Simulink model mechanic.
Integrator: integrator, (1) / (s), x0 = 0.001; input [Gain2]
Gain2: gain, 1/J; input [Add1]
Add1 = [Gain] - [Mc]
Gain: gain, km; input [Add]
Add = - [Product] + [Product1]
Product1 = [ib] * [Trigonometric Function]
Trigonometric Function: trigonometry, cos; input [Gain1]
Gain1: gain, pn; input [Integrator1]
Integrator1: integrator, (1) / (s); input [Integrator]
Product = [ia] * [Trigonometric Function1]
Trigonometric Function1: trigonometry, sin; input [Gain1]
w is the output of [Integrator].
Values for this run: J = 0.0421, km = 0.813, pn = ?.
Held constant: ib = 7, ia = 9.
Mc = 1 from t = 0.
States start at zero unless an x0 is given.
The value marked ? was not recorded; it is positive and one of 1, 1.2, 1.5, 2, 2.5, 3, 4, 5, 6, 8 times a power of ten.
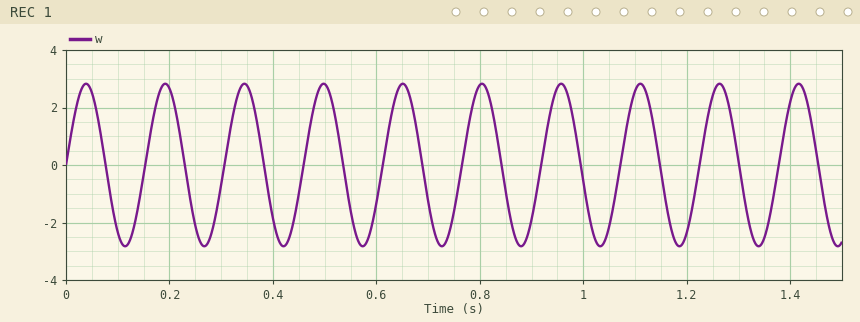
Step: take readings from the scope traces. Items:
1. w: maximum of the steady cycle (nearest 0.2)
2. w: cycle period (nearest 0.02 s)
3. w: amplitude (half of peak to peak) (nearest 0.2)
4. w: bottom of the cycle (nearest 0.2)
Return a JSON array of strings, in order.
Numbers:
["2.8", "0.16 s", "2.8", "-2.8"]
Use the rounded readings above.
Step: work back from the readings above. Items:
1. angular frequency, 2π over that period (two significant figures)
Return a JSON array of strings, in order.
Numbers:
["39 rad/s"]
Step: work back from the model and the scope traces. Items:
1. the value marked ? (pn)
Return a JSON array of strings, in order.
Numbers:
["8"]
